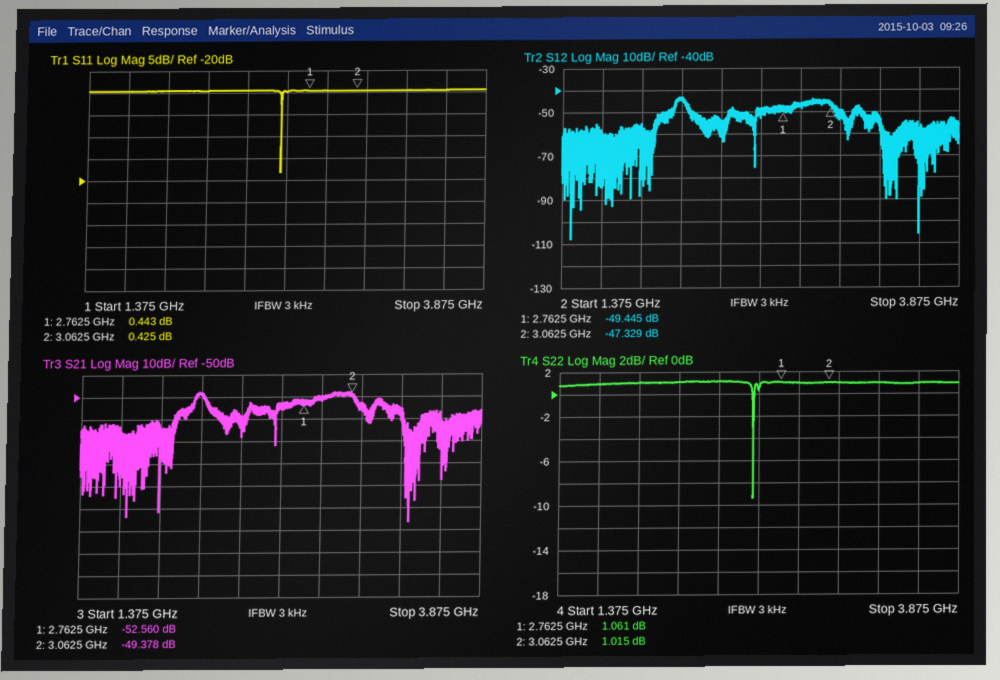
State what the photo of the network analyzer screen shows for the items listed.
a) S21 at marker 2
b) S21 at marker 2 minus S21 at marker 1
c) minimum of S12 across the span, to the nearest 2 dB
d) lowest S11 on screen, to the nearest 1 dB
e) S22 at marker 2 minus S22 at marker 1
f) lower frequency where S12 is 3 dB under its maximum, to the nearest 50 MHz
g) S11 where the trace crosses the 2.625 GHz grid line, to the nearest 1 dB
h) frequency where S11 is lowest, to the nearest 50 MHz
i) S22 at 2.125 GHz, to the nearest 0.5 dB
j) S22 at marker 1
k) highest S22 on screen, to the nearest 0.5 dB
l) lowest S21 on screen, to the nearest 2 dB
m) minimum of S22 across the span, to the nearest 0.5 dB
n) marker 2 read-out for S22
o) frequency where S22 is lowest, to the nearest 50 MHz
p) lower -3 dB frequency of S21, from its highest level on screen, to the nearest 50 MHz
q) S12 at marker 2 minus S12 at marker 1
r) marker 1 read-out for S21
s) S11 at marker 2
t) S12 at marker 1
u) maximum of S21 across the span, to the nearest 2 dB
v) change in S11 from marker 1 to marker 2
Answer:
-49.378 dB
3.182 dB
-108 dB
-18 dB
-0.046 dB
2.10 GHz
0 dB
2.60 GHz
1.0 dB
1.061 dB
1.0 dB
-106 dB
-9.5 dB
1.015 dB
2.60 GHz
2.10 GHz
2.116 dB
-52.560 dB
0.425 dB
-49.445 dB
-48 dB
-0.018 dB
